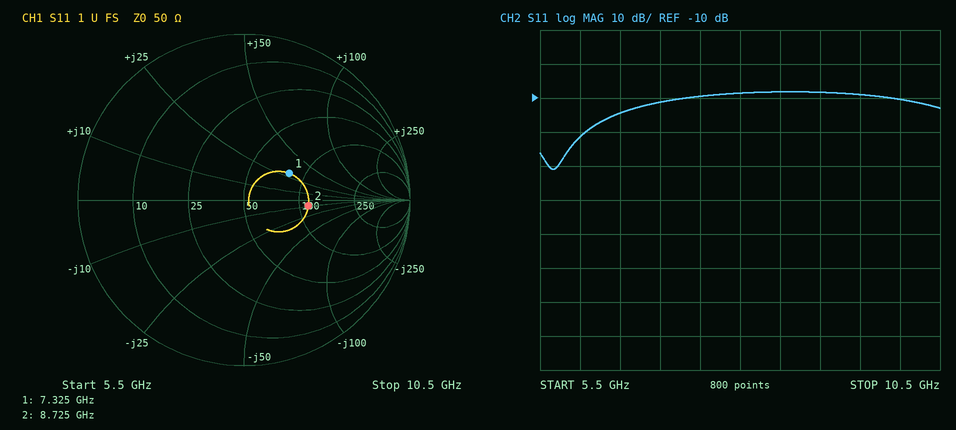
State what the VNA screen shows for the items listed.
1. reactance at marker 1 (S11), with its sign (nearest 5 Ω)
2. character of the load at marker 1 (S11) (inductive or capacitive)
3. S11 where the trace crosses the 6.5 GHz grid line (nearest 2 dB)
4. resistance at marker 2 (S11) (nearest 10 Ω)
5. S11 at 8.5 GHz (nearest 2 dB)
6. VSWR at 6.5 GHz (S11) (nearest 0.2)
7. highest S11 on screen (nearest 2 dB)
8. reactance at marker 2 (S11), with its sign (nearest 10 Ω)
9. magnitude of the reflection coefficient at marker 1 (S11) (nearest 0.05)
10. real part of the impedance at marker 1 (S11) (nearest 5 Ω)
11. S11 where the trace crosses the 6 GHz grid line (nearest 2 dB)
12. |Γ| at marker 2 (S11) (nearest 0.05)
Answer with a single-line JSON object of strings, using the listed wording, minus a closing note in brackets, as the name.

{"reactance at marker 1 (S11), with its sign": "+30 Ω", "character of the load at marker 1 (S11)": "inductive", "S11 where the trace crosses the 6.5 GHz grid line": "-14 dB", "resistance at marker 2 (S11)": "110 Ω", "S11 at 8.5 GHz": "-8 dB", "VSWR at 6.5 GHz (S11)": "1.4", "highest S11 on screen": "-8 dB", "reactance at marker 2 (S11), with its sign": "-10 Ω", "magnitude of the reflection coefficient at marker 1 (S11)": "0.30", "real part of the impedance at marker 1 (S11)": "80 Ω", "S11 where the trace crosses the 6 GHz grid line": "-22 dB", "|Γ| at marker 2 (S11)": "0.40"}
